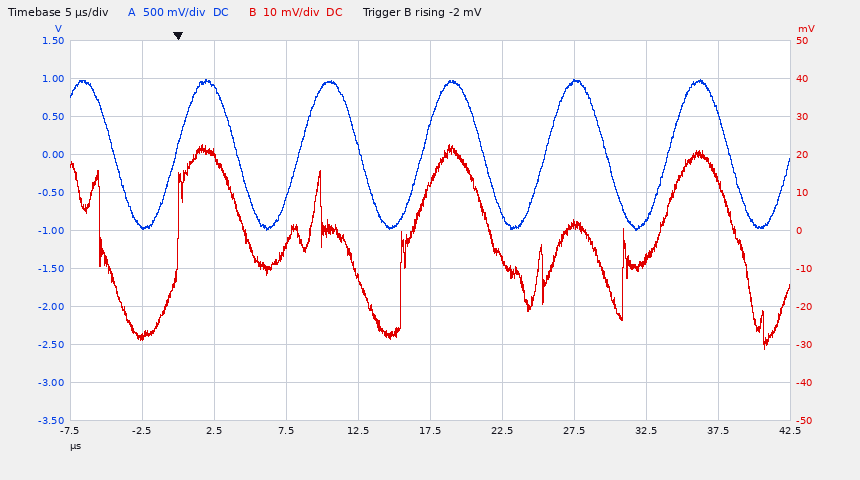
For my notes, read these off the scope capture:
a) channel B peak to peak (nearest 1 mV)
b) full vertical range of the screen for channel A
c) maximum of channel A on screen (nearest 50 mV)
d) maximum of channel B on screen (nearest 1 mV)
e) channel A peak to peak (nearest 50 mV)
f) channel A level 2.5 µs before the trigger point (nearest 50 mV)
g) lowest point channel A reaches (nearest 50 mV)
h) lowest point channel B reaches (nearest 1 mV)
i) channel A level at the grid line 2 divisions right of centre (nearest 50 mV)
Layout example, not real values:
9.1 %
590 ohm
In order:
54 mV
5 V
1.00 V
23 mV
2.00 V
-950 mV
-1.00 V
-31 mV
950 mV
